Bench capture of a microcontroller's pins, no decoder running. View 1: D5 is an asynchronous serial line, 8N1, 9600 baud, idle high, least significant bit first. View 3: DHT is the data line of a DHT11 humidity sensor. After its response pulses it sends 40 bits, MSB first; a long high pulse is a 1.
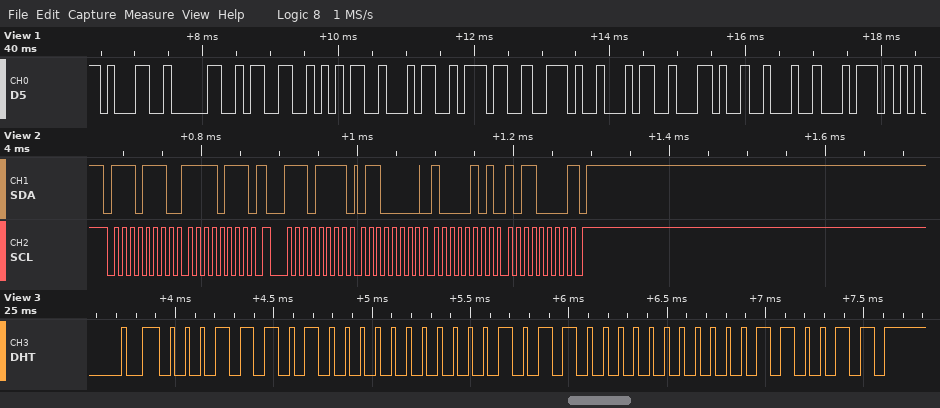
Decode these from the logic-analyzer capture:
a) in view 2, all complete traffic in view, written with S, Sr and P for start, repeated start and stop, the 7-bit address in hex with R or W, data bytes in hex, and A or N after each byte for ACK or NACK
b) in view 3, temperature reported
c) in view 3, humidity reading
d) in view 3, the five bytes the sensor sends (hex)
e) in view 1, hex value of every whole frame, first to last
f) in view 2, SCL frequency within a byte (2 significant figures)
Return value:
S 77W A F7 A Sr 77R A 60 A 85 A B0 N P
22.0 °C
29 %
1D 00 16 00 33
31 30 33 35 34 37 2E 34 2C 22 74
100 kHz
